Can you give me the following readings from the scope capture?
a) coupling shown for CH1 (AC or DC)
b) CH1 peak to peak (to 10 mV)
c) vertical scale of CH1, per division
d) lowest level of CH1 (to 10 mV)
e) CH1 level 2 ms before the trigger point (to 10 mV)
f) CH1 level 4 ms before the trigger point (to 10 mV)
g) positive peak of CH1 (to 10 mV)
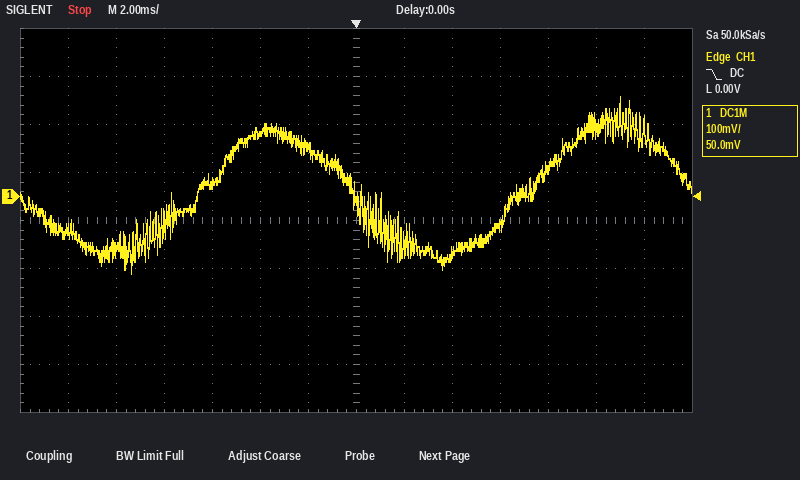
DC
370 mV
100 mV
-160 mV
100 mV
130 mV
210 mV
